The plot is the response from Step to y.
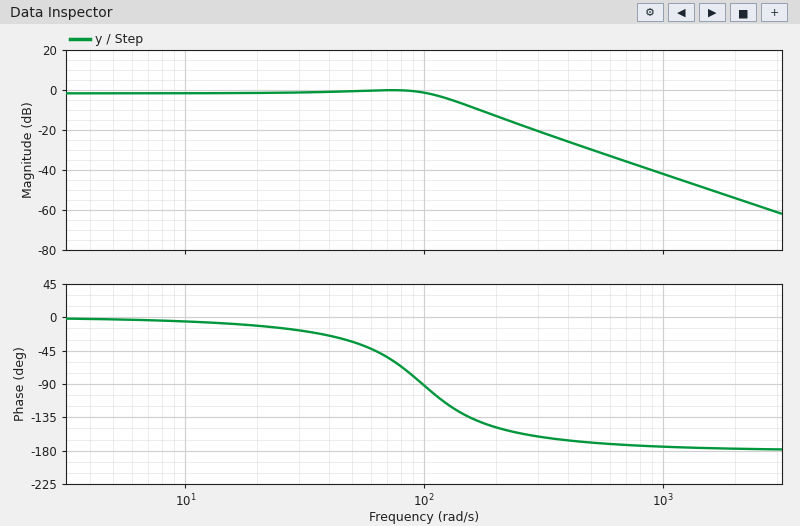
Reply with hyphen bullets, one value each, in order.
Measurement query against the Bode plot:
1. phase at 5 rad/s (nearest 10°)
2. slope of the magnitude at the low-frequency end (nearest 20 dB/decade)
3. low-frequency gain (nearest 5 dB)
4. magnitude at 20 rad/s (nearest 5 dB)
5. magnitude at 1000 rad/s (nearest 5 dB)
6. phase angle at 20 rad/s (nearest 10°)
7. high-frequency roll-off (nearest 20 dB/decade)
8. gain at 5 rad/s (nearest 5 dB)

- 0°
- 0 dB/decade
- 0 dB
- 0 dB
- -40 dB
- -10°
- -40 dB/decade
- 0 dB
